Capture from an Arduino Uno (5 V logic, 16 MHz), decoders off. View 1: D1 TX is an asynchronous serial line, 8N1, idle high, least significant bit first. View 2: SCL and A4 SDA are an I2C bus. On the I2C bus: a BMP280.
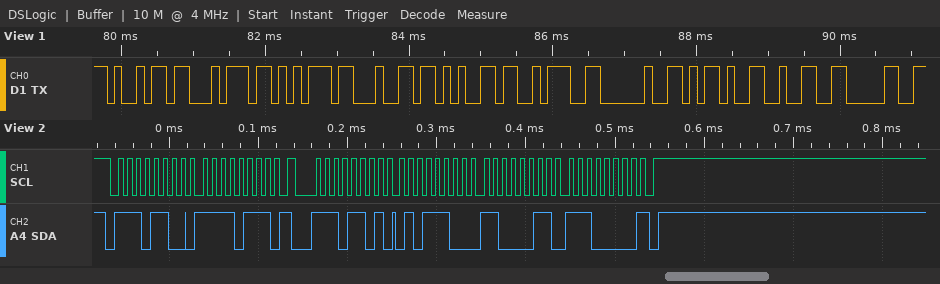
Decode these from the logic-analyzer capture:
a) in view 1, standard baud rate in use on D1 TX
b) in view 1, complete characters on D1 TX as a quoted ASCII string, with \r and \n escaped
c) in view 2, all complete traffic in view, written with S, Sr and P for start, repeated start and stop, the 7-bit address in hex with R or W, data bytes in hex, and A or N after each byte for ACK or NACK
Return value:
9600 baud
"itude: -20"
S 76W A F7 A Sr 76R A 5C A C3 A E0 N P
